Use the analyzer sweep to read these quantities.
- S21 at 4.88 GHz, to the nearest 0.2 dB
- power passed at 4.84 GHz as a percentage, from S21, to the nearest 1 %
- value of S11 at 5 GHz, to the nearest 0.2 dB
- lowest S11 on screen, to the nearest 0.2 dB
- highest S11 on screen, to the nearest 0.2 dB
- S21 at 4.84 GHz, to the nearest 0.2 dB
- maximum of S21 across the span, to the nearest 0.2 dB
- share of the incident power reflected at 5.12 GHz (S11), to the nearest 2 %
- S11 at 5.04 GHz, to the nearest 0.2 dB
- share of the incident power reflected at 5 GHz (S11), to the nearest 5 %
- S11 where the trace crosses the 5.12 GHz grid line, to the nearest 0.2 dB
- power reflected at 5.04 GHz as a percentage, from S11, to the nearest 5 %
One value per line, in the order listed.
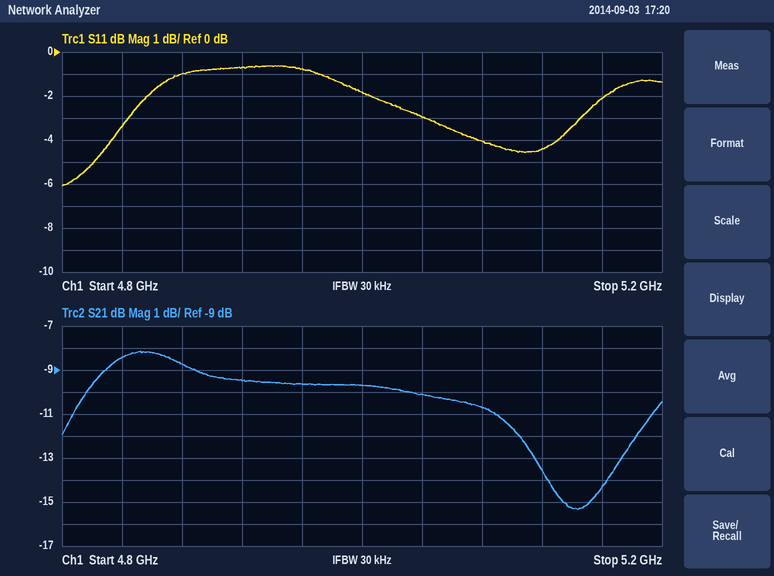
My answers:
-8.8 dB
14 %
-1.8 dB
-6.0 dB
-0.6 dB
-8.4 dB
-8.2 dB
36 %
-3.0 dB
65 %
-4.4 dB
50 %
